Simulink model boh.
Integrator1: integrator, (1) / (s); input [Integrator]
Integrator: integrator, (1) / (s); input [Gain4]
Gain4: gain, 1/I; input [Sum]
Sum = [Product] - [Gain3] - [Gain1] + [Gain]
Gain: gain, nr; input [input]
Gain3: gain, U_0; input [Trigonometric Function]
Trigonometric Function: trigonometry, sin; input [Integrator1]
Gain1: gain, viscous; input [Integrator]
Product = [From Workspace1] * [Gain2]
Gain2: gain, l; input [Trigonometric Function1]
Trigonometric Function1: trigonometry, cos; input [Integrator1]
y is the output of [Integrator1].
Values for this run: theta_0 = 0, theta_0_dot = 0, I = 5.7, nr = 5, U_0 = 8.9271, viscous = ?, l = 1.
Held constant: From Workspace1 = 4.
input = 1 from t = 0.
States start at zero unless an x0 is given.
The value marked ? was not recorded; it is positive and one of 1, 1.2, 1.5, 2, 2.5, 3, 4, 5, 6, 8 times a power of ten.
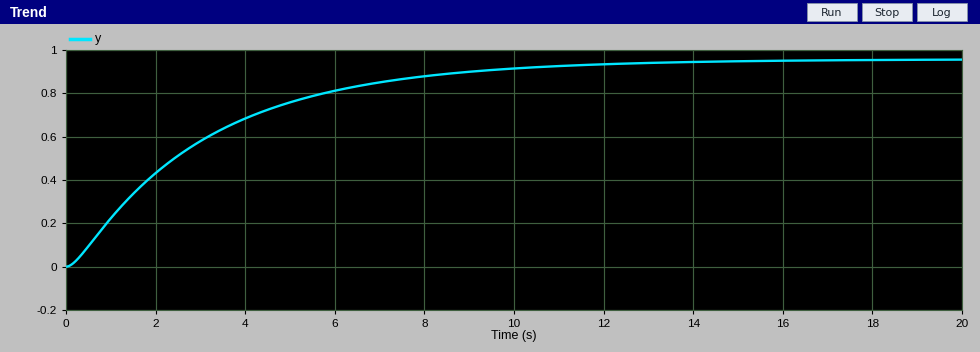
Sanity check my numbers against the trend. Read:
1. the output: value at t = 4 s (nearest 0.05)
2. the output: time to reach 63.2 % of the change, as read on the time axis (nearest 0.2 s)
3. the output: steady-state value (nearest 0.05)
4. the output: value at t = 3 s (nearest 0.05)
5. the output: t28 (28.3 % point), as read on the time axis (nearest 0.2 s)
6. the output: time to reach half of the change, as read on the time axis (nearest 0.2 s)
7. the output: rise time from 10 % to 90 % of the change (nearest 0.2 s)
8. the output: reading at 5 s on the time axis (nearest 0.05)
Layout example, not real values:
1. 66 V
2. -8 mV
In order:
1. 0.70
2. 3.2 s
3. 0.95
4. 0.60
5. 1.2 s
6. 2.2 s
7. 6.8 s
8. 0.75
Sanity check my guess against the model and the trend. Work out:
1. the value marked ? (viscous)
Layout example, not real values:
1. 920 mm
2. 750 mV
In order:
1. 30
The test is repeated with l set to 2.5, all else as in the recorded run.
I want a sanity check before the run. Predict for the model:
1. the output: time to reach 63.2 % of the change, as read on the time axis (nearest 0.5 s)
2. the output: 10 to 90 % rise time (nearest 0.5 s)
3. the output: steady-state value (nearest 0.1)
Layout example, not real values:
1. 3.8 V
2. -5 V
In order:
1. 2.5 s
2. 4.5 s
3. 1.2
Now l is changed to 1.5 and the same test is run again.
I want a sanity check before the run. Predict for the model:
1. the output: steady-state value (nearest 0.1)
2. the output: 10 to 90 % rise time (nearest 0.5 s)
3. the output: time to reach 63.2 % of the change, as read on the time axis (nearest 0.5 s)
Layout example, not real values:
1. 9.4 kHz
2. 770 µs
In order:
1. 1.1
2. 6.0 s
3. 3.0 s
